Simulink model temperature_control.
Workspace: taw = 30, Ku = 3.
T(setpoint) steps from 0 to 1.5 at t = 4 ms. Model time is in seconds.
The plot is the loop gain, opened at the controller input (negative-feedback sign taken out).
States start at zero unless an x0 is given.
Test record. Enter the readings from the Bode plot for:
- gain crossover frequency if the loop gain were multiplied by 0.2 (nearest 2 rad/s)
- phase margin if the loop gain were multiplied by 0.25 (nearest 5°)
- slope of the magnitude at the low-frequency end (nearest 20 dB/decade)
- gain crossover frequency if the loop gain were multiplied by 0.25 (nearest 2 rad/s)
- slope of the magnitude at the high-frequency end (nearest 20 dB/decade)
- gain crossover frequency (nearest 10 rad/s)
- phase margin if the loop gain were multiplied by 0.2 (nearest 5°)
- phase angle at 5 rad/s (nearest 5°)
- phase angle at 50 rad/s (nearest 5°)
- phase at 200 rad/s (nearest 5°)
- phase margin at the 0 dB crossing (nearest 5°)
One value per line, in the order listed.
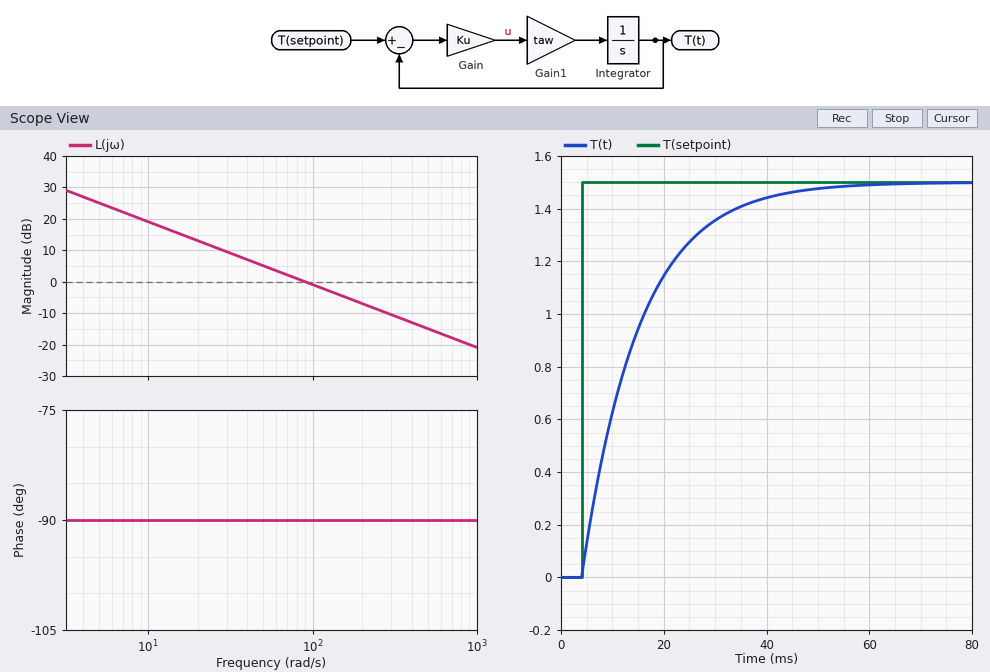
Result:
18 rad/s
90°
-20 dB/decade
22 rad/s
-20 dB/decade
90 rad/s
90°
-90°
-90°
-90°
90°
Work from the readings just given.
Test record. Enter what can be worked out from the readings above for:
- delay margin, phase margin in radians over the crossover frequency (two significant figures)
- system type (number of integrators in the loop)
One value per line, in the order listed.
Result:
0.017 s
1
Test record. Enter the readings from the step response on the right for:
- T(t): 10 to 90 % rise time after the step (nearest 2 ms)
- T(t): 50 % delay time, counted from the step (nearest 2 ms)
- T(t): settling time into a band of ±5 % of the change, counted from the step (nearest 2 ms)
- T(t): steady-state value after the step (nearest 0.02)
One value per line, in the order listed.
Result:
24 ms
8 ms
34 ms
1.50
